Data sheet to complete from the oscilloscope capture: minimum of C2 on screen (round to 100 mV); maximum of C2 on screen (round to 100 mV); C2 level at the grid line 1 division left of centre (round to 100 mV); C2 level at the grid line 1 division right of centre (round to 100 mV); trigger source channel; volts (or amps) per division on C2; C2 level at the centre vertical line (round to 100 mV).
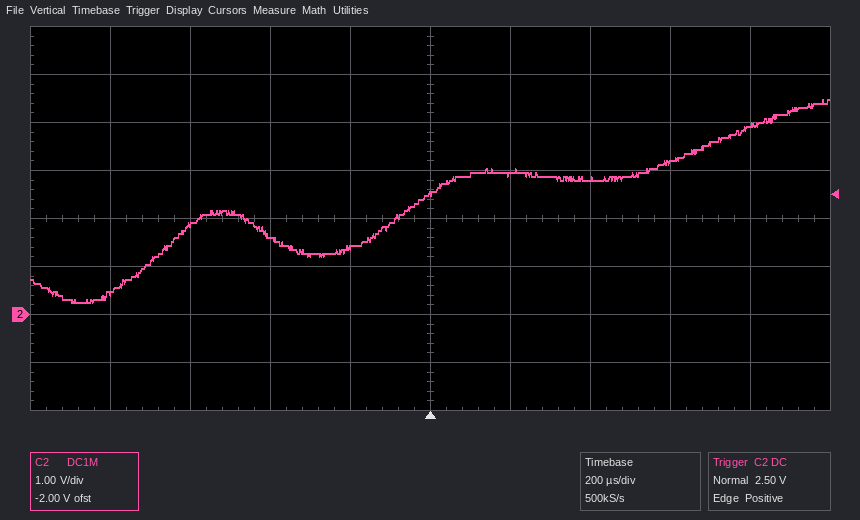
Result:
200 mV
4.5 V
1.4 V
2.9 V
C2
1 V
2.5 V
